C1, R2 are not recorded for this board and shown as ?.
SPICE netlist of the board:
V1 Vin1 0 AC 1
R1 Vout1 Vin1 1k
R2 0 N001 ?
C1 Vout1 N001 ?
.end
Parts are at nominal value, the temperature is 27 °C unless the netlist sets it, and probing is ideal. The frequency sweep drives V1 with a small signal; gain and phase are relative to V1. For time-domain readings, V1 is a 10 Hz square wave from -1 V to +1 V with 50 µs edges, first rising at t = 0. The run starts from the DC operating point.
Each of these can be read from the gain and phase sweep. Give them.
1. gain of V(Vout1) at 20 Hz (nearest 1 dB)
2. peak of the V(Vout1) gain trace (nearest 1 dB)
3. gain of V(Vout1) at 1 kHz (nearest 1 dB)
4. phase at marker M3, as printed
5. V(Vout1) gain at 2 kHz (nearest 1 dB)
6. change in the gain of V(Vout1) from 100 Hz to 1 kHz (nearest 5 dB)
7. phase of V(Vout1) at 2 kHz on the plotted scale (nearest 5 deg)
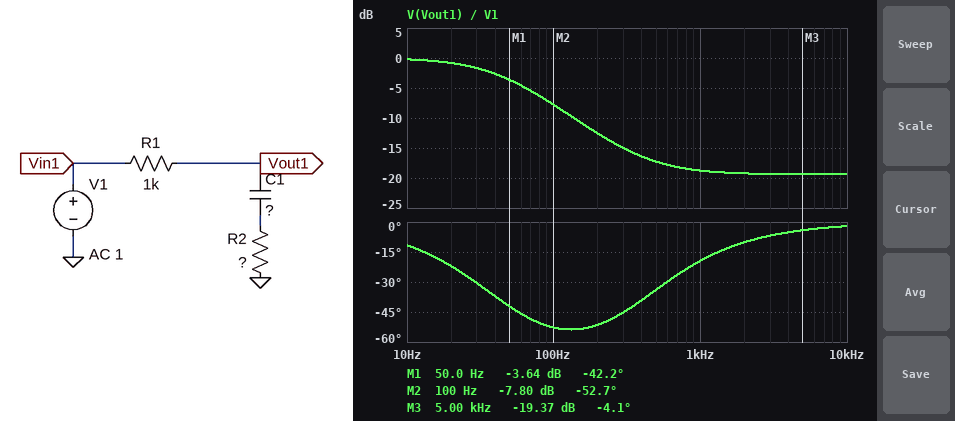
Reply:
-1 dB
0 dB
-19 dB
-4.1 deg
-19 dB
-10 dB
-10 deg
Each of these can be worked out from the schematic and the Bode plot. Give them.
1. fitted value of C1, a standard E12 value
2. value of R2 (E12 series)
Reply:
3.3 µF
120 Ω
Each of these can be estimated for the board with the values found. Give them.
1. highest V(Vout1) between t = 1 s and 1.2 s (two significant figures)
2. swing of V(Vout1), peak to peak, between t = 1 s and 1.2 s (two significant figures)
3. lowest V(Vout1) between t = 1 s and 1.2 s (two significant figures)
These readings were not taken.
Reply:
1.0 V
2.0 V
-1.0 V
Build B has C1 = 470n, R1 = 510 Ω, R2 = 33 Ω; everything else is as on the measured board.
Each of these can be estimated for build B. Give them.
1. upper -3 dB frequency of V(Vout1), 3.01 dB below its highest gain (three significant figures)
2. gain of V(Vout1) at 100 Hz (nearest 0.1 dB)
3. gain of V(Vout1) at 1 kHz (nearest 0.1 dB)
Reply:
626 Hz
-0.1 dB
-5.5 dB
